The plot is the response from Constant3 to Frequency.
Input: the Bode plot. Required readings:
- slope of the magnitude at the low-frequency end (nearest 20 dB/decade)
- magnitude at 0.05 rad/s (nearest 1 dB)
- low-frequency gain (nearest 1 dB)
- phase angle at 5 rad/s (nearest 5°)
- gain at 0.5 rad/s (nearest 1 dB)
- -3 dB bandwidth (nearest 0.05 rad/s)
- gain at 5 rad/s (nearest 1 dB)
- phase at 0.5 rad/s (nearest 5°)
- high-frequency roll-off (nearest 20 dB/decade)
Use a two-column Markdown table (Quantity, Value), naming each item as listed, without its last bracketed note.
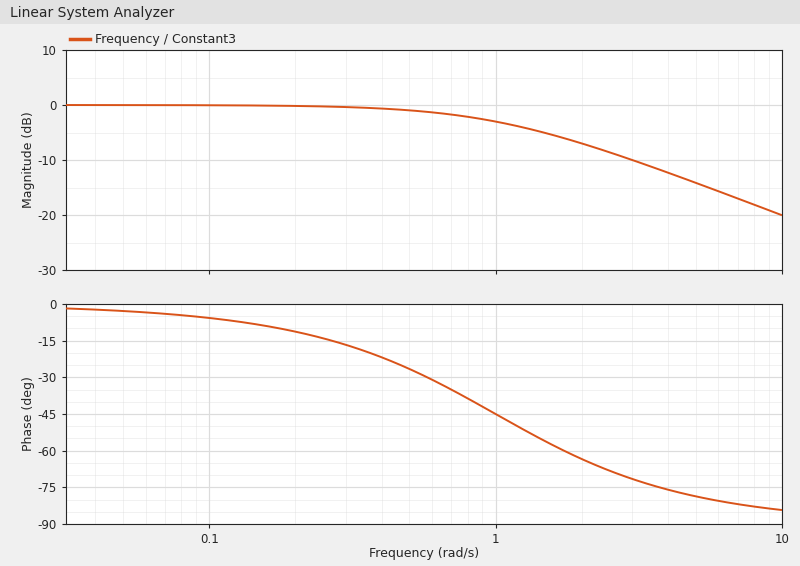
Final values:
| Quantity | Value |
|---|---|
| slope of the magnitude at the low-frequency end | 0 dB/decade |
| magnitude at 0.05 rad/s | 0 dB |
| low-frequency gain | 0 dB |
| phase angle at 5 rad/s | -80° |
| gain at 0.5 rad/s | -1 dB |
| -3 dB bandwidth | 1.00 rad/s |
| gain at 5 rad/s | -14 dB |
| phase at 0.5 rad/s | -25° |
| high-frequency roll-off | -20 dB/decade |
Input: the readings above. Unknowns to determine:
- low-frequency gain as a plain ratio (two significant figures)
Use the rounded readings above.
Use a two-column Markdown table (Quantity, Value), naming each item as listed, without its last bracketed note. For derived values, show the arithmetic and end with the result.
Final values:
| Quantity | Value |
|---|---|
| low-frequency gain as a plain ratio | 10^(0 / 20) = 1.0 |
